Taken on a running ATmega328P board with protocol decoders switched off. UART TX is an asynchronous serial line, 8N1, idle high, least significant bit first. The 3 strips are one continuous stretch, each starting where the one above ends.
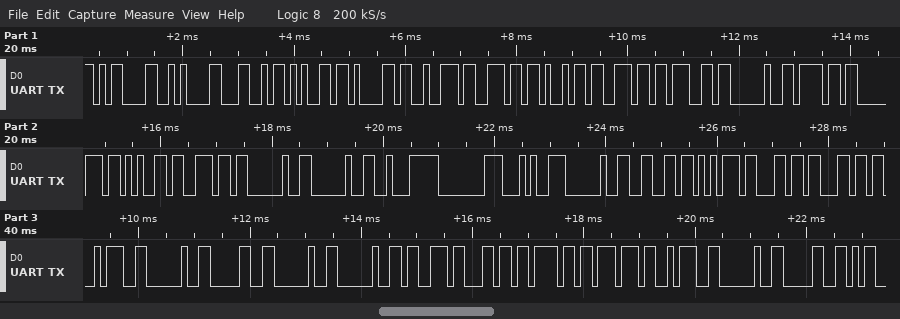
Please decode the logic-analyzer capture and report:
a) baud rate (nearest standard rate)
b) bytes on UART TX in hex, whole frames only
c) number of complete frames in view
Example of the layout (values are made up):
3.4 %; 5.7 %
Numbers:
9600 baud; 0D 0A 4C 65 61 72 6E 69 6E 67 20 6F 70 65 6E 20 20 E2 80 94 20 66 75 6C 6C 3A 20 30 20 20 73 6C 6F 77 3A 20 30; 37
